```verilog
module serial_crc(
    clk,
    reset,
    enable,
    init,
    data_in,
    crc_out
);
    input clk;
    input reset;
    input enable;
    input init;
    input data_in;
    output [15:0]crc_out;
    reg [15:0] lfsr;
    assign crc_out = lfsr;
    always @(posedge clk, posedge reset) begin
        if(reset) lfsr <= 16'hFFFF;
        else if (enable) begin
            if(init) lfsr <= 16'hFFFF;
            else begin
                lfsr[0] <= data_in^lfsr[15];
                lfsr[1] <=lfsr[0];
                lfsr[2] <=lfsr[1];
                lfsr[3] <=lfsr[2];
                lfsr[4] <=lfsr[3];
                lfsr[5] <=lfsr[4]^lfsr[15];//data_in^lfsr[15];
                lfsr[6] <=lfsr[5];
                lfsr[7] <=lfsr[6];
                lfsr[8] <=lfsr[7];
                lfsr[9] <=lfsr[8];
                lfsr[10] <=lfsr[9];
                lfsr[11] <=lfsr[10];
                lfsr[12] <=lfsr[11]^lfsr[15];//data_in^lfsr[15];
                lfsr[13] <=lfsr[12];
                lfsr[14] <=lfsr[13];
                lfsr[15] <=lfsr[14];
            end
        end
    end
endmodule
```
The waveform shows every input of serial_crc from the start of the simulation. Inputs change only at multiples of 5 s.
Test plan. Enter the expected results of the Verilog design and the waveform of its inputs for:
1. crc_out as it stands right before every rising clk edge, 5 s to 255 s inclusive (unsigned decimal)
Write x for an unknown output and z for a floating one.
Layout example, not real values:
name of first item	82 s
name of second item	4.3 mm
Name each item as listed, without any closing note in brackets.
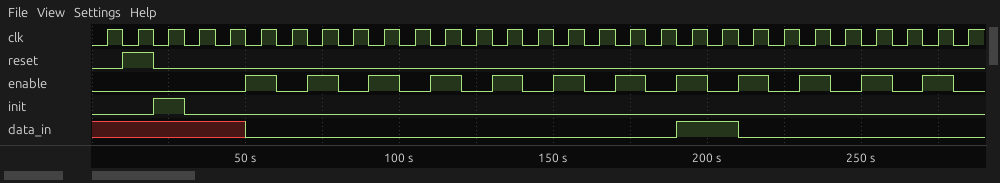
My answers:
crc_out as it stands right before every rising clk edge, 5 s to 255 s inclusive	x, 65535, 65535, 65535, 65535, 65535, 61407, 61407, 53151, 53151, 36639, 36639, 3615, 3615, 7230, 7230, 14460, 14460, 28920, 28920, 57841, 57841, 54211, 54211, 47015, 47015
